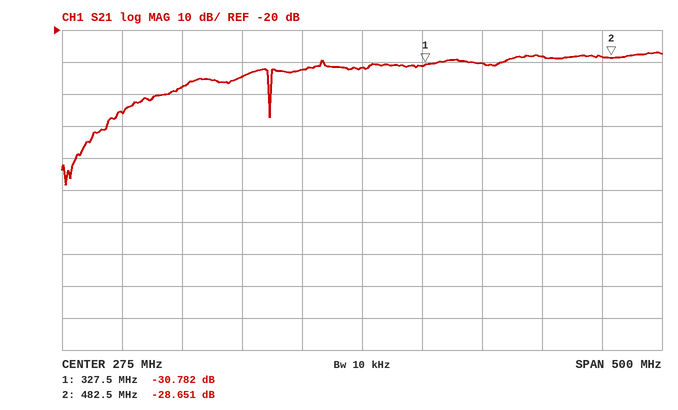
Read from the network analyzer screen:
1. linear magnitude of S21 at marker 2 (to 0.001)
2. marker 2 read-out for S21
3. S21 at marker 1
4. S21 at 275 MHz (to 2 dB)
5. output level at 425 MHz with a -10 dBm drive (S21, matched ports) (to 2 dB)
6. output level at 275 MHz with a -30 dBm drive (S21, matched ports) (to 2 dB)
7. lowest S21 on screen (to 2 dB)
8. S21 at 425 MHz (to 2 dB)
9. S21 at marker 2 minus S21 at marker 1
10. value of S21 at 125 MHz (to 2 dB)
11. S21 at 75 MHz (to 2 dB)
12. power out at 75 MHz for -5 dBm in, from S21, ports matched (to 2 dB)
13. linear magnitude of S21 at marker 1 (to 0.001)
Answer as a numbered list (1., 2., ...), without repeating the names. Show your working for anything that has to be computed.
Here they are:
1. 10^(-28.651/20) ≈ 0.037
2. -28.651 dB
3. -30.782 dB
4. -32 dB
5. -10 dBm + (-28 dB) = -38 dBm
6. -30 dBm + (-32 dB) = -62 dBm
7. -68 dB
8. -28 dB
9. -28.651 − (-30.782) = 2.131 dB
10. -38 dB
11. -46 dB
12. -5 dBm + (-46 dB) = -50 dBm
13. 10^(-30.782/20) ≈ 0.029
